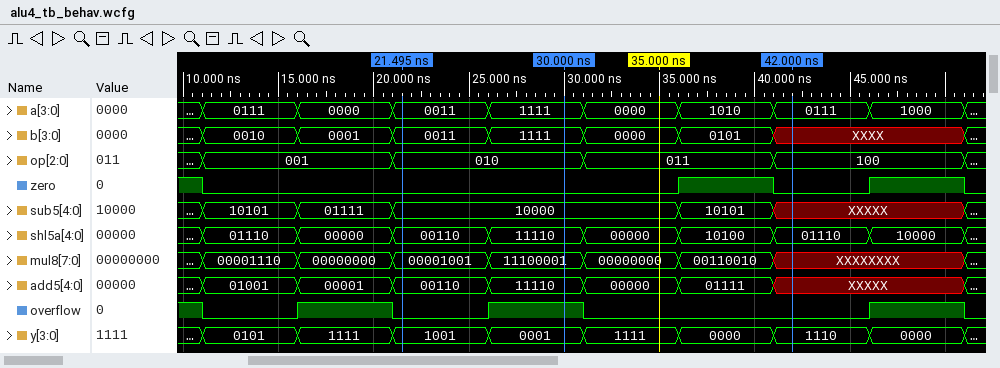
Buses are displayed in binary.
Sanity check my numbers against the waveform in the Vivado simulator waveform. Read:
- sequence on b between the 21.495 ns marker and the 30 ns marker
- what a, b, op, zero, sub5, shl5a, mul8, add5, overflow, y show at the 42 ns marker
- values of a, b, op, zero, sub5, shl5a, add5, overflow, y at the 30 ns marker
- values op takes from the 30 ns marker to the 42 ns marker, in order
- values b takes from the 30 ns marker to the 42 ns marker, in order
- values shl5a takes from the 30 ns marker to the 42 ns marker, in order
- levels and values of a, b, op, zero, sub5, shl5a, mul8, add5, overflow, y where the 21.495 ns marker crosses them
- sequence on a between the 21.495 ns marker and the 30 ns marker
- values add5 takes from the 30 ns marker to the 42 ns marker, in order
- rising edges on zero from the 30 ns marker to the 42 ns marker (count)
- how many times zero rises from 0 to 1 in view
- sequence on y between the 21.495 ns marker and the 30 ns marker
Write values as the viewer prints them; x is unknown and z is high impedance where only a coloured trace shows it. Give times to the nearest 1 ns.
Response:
0011, 1111
a=0111, b=XXXX, op=100, zero=0, sub5=XXXXX, shl5a=01110, mul8=XXXXXXXX, add5=XXXXX, overflow=0, y=1110
a=1111, b=1111, op=010, zero=0, sub5=10000, shl5a=11110, add5=11110, overflow=1, y=0001
010, 011, 100
1111, 0000, 0101, XXXX
11110, 00000, 10100, 01110
a=0011, b=0011, op=010, zero=0, sub5=10000, shl5a=00110, mul8=00001001, add5=00110, overflow=0, y=1001
0011, 1111
11110, 00000, 01111, XXXXX
1
2
1001, 0001
